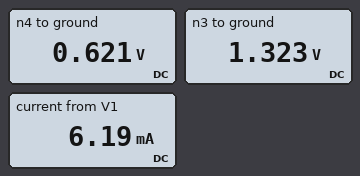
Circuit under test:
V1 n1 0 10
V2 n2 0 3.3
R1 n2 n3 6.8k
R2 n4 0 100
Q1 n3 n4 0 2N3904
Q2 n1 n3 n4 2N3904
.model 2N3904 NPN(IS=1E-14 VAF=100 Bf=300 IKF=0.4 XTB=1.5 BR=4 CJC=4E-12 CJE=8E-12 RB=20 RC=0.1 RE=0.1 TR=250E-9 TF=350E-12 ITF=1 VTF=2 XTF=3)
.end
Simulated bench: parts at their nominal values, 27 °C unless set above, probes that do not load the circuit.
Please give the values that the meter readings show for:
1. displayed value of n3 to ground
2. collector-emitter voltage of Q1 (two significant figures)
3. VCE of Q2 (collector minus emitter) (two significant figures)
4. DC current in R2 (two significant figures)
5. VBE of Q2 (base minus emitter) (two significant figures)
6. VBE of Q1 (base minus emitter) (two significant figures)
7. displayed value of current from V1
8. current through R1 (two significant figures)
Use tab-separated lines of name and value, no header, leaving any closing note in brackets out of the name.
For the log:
displayed value of n3 to ground	1.323 V
collector-emitter voltage of Q1	1.3 V
VCE of Q2 (collector minus emitter)	9.4 V
DC current in R2	6.2 mA
VBE of Q2 (base minus emitter)	700 mV
VBE of Q1 (base minus emitter)	620 mV
displayed value of current from V1	6.19 mA
current through R1	290 µA
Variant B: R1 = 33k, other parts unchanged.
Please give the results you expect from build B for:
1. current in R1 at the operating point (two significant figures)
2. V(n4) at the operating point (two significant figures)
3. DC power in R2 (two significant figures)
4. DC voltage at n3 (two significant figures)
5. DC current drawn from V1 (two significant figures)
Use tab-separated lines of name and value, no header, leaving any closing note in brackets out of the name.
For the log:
current in R1 at the operating point	61 µA
V(n4) at the operating point	570 mV
DC power in R2	3.3 mW
DC voltage at n3	1.3 V
DC current drawn from V1	5.7 mA
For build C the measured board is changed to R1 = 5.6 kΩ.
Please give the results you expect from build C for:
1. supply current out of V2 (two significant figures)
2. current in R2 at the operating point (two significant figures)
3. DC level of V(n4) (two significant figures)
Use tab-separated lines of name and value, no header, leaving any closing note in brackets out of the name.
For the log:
supply current out of V2	350 µA
current in R2 at the operating point	6.3 mA
DC level of V(n4)	630 mV
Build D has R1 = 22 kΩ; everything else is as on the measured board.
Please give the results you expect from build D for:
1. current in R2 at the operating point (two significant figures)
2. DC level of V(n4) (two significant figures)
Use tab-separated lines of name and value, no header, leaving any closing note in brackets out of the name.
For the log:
current in R2 at the operating point	5.9 mA
DC level of V(n4)	590 mV
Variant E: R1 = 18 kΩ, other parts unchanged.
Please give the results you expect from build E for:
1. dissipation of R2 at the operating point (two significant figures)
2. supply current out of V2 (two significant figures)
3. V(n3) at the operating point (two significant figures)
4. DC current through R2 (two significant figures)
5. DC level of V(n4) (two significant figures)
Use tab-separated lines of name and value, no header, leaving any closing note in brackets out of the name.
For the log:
dissipation of R2 at the operating point	3.5 mW
supply current out of V2	110 µA
V(n3) at the operating point	1.3 V
DC current through R2	5.9 mA
DC level of V(n4)	590 mV
